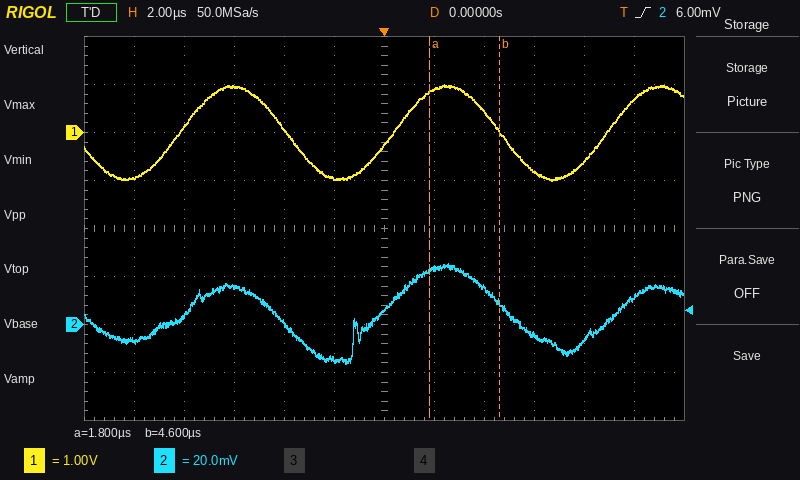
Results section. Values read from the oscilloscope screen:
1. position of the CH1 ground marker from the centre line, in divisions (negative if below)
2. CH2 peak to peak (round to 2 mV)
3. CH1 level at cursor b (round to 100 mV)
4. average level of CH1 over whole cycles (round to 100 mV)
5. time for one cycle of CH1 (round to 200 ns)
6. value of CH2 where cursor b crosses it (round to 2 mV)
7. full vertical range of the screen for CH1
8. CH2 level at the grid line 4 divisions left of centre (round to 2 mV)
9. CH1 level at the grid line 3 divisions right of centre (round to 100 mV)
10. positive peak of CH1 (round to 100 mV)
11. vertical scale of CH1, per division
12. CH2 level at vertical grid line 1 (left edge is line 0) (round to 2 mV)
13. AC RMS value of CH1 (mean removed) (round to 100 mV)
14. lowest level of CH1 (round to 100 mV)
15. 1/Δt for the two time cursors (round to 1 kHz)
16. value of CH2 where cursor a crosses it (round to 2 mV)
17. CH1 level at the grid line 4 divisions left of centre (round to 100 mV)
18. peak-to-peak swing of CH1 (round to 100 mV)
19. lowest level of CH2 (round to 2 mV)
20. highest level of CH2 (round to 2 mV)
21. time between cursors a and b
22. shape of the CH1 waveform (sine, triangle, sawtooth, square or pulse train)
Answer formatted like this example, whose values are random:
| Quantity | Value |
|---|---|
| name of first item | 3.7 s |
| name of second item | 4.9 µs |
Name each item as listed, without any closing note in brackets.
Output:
| Quantity | Value |
|---|---|
| position of the CH1 ground marker from the centre line, in divisions | +2.0 div |
| CH2 peak to peak | 42 mV |
| CH1 level at cursor b | 0.0 V |
| average level of CH1 over whole cycles | 0.0 V |
| time for one cycle of CH1 | 8.6 µs |
| value of CH2 where cursor b crosses it | 8 mV |
| full vertical range of the screen for CH1 | 8 V |
| CH2 level at the grid line 4 divisions left of centre | 4 mV |
| CH1 level at the grid line 3 divisions right of centre | -800 mV |
| positive peak of CH1 | 1.0 V |
| vertical scale of CH1, per division | 1 V |
| CH2 level at vertical grid line 1 (left edge is line 0) | -6 mV |
| AC RMS value of CH1 (mean removed) | 700 mV |
| lowest level of CH1 | -1.0 V |
| 1/Δt for the two time cursors | 357 kHz |
| value of CH2 where cursor a crosses it | 22 mV |
| CH1 level at the grid line 4 divisions left of centre | 100 mV |
| peak-to-peak swing of CH1 | 2.0 V |
| lowest level of CH2 | -16 mV |
| highest level of CH2 | 26 mV |
| time between cursors a and b | 2.8 µs |
| shape of the CH1 waveform | sine |
